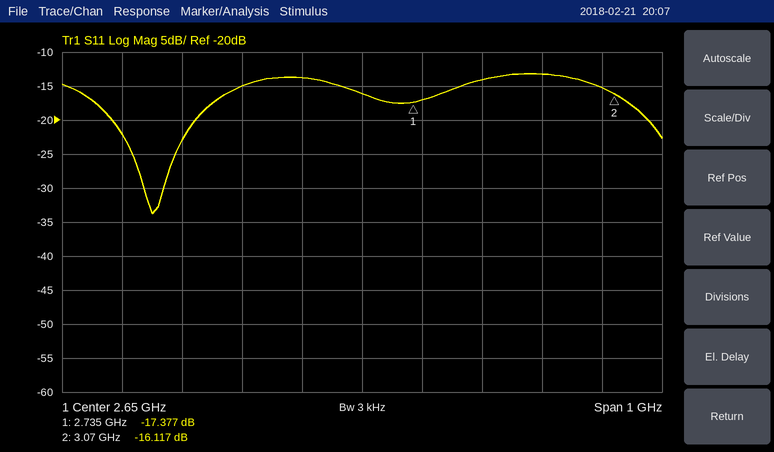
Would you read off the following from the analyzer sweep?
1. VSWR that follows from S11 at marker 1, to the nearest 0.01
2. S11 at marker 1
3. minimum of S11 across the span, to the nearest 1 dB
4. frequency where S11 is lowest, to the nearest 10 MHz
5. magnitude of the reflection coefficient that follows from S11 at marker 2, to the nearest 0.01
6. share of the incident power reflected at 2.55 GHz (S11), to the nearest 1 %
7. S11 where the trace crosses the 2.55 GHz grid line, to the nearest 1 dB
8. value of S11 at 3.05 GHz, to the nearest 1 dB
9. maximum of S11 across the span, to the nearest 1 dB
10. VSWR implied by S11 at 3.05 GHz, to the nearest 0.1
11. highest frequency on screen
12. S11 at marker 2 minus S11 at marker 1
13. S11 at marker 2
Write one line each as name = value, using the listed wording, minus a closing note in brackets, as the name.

VSWR that follows from S11 at marker 1, to the nearest 0.01 = 1.31
S11 at marker 1 = -17.377 dB
minimum of S11 across the span, to the nearest 1 dB = -34 dB
frequency where S11 is lowest, to the nearest 10 MHz = 2.30 GHz
magnitude of the reflection coefficient that follows from S11 at marker 2, to the nearest 0.01 = 0.16
share of the incident power reflected at 2.55 GHz (S11), to the nearest 1 % = 4 %
S11 where the trace crosses the 2.55 GHz grid line, to the nearest 1 dB = -14 dB
value of S11 at 3.05 GHz, to the nearest 1 dB = -15 dB
maximum of S11 across the span, to the nearest 1 dB = -13 dB
VSWR implied by S11 at 3.05 GHz, to the nearest 0.1 = 1.4
highest frequency on screen = 3.15 GHz
S11 at marker 2 minus S11 at marker 1 = 1.260 dB
S11 at marker 2 = -16.117 dB
